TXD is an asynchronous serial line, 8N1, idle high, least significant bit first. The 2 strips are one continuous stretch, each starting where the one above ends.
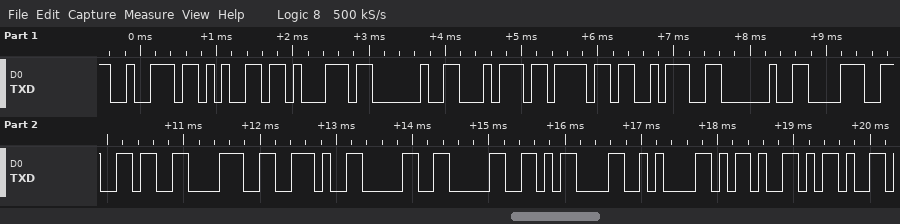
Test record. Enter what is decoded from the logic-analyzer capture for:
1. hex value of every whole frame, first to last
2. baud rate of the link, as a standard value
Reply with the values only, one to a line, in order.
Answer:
72 65 71 20 74 6F 3A 20 38 36 38 2E 30 30 0D 0A 2D 2D
9600 baud
